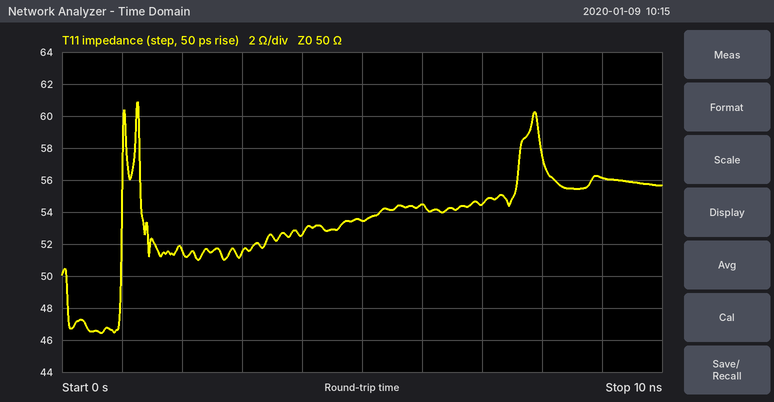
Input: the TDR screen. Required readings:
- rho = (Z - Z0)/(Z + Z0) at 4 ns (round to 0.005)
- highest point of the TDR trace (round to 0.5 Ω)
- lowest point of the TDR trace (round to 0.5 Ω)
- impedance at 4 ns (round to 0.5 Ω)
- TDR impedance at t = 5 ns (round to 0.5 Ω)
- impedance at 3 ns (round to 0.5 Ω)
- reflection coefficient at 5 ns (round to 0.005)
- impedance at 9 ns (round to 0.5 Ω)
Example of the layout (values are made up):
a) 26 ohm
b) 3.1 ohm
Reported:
a) +0.025
b) 61.0 Ω
c) 46.5 Ω
d) 52.5 Ω
e) 53.5 Ω
f) 51.5 Ω
g) +0.035
h) 56.0 Ω
